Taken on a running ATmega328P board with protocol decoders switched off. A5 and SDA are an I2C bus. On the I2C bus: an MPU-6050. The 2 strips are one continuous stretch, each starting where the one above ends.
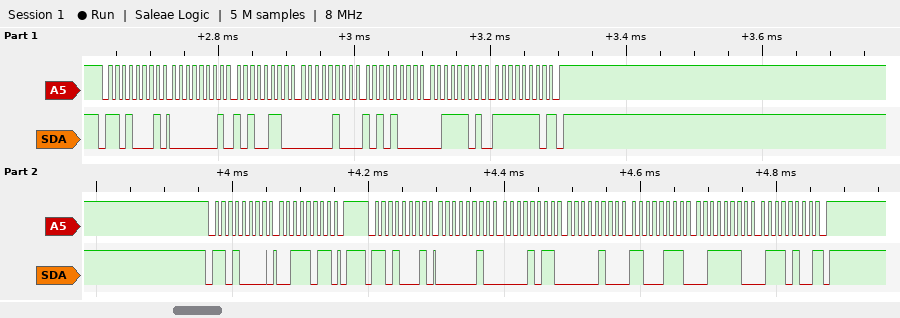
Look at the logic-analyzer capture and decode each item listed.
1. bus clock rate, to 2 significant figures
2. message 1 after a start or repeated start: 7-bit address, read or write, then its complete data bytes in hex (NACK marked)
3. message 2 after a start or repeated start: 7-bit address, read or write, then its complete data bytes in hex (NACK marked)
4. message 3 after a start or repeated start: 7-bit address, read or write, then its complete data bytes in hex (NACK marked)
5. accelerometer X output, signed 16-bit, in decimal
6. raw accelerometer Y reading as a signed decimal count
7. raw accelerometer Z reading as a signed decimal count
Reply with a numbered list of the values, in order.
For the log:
1. 100 kHz
2. 0x68 read: 01 A6 04 A8 3D FE NACK
3. 0x68 write: 3B
4. 0x68 read: 02 0B 04 C7 3E 74 NACK
5. 523
6. 1223
7. 15988
